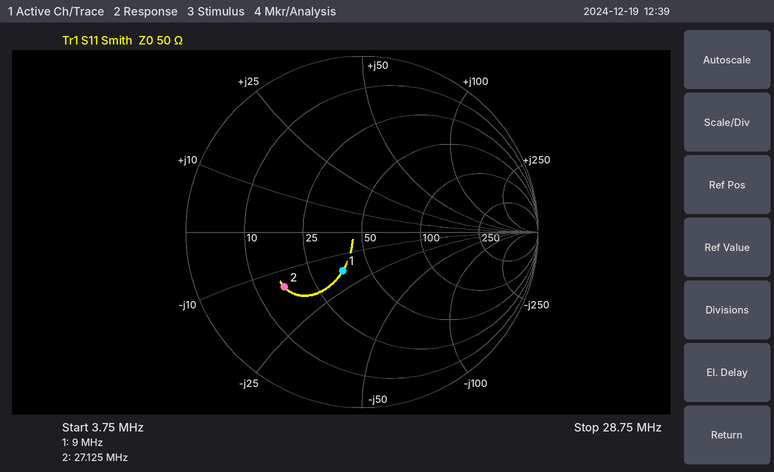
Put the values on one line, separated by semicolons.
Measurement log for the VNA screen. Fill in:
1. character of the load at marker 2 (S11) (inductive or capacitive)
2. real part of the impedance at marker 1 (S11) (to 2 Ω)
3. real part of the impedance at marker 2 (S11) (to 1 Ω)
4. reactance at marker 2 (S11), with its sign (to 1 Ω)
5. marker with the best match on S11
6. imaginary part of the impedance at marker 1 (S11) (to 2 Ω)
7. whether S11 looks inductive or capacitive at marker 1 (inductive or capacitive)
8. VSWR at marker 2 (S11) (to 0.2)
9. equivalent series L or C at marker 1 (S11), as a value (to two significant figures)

capacitive; 36 Ω; 16 Ω; -14 Ω; marker 1; -18 Ω; capacitive; 3.4; 1.0 nF
